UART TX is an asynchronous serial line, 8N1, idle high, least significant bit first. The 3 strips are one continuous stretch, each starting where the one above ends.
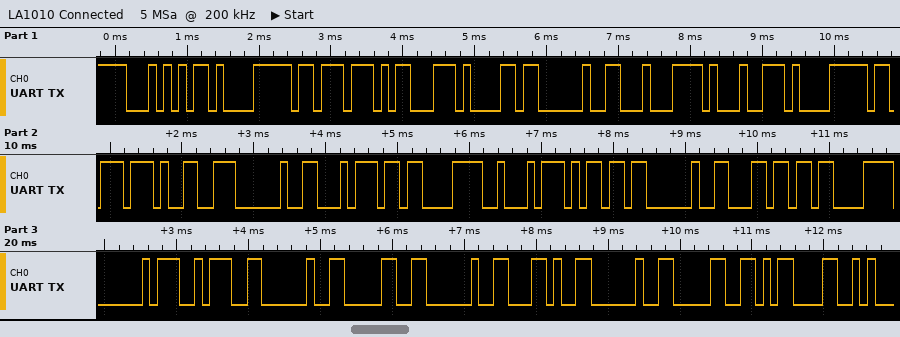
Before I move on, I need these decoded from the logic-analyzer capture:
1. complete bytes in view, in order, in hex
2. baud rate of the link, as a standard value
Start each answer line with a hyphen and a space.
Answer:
- 0x54 0xE1 0xBB 0x8D 0x61 0x20 0xC4 0x91 0xE1 0xBB 0x99 0x20 0x74 0xC3 0xA2 0x6D 0x20 0x6C 0xC3 0xA0 0x3A 0x20 0x30 0x20 0x2C 0x20 0x30 0x0D
- 9600 baud
